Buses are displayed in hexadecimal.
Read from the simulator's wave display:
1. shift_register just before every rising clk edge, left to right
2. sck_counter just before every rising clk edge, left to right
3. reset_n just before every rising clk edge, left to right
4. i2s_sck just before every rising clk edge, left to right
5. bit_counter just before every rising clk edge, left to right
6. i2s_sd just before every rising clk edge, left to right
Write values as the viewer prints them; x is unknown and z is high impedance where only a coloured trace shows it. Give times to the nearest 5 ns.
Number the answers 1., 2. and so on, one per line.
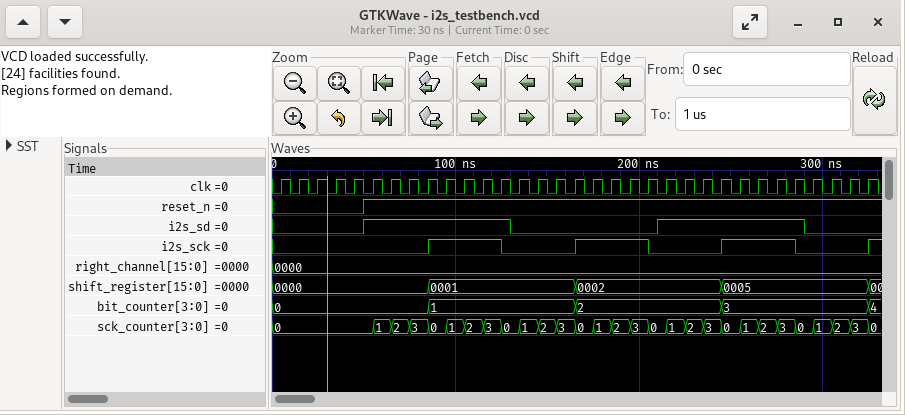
1. 0000, 0000, 0000, 0000, 0000, 0000, 0000, 0000, 0000, 0001, 0001, 0001, 0001, 0001, 0001, 0001, 0001, 0002, 0002, 0002, 0002, 0002, 0002, 0002, 0002, 0005, 0005, 0005, 0005, 0005, 0005, 0005, 0005
2. 0, 0, 0, 0, 0, 0, 1, 2, 3, 0, 1, 2, 3, 0, 1, 2, 3, 0, 1, 2, 3, 0, 1, 2, 3, 0, 1, 2, 3, 0, 1, 2, 3
3. 0 0 0 0 0 1 1 1 1 1 1 1 1 1 1 1 1 1 1 1 1 1 1 1 1 1 1 1 1 1 1 1 1
4. 0 0 0 0 0 0 0 0 0 1 1 1 1 0 0 0 0 1 1 1 1 0 0 0 0 1 1 1 1 0 0 0 0
5. 0, 0, 0, 0, 0, 0, 0, 0, 0, 1, 1, 1, 1, 1, 1, 1, 1, 2, 2, 2, 2, 2, 2, 2, 2, 3, 3, 3, 3, 3, 3, 3, 3
6. 0 0 0 0 0 1 1 1 1 1 1 1 1 0 0 0 0 0 0 0 0 1 1 1 1 1 1 1 1 0 0 0 0
